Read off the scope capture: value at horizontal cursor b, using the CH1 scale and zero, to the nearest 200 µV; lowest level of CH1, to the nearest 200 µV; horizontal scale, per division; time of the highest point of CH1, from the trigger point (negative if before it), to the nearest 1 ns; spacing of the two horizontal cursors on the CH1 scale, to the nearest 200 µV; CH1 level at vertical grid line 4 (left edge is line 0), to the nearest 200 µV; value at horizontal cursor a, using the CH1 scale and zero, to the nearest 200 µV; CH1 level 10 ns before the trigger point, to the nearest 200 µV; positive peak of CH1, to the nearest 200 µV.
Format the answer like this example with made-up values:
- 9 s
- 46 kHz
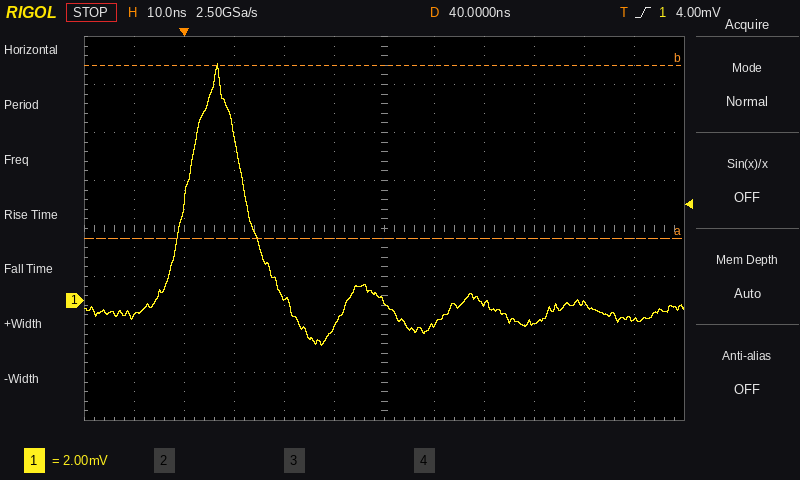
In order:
- 9.8 mV
- -1.8 mV
- 10 ns
- +7 ns
- 7.2 mV
- 200 µV
- 2.6 mV
- -600 µV
- 9.8 mV
